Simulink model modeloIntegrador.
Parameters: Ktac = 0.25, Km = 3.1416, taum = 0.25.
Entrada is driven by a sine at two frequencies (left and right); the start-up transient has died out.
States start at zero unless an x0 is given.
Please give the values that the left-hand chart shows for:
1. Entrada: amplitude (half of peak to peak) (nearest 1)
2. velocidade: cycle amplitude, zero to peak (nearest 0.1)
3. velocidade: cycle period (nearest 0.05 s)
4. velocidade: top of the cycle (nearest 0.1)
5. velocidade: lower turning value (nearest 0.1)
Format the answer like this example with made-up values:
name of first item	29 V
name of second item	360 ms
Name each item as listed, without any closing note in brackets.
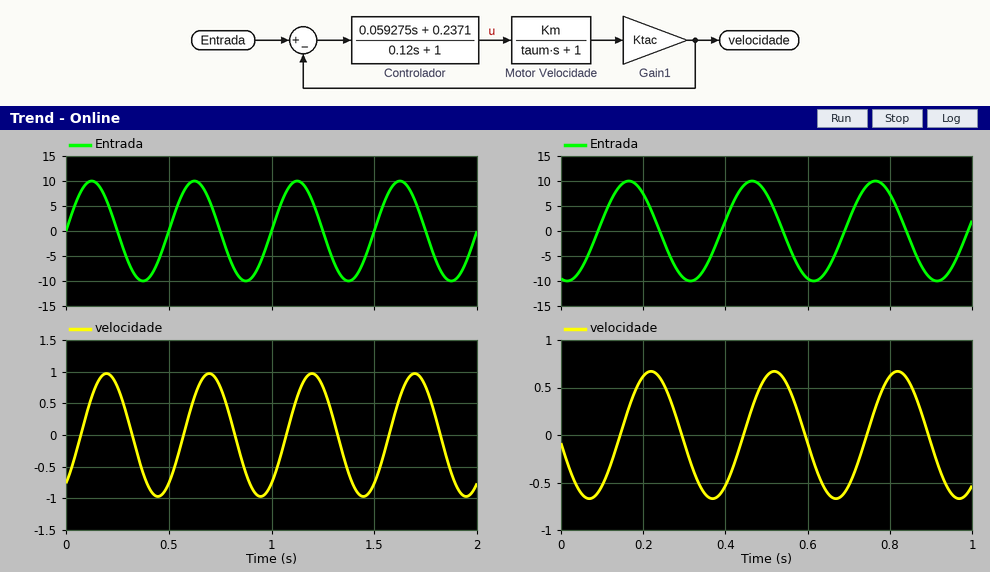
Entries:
Entrada: amplitude (half of peak to peak)	10
velocidade: cycle amplitude, zero to peak	1.0
velocidade: cycle period	0.50 s
velocidade: top of the cycle	1.0
velocidade: lower turning value	-1.0
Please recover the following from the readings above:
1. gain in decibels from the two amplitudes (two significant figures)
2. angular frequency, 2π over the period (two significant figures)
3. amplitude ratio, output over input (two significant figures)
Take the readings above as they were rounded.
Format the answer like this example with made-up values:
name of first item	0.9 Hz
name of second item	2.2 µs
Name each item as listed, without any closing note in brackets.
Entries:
gain in decibels from the two amplitudes	-20 dB
angular frequency, 2π over the period	13 rad/s
amplitude ratio, output over input	0.10
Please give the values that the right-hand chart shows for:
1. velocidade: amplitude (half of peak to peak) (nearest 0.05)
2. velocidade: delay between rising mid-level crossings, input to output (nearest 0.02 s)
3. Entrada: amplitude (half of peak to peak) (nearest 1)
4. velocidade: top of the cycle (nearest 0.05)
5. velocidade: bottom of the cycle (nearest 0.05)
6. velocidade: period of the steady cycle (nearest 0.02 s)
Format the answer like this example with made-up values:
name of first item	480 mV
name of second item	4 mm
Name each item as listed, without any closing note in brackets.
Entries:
velocidade: amplitude (half of peak to peak)	0.65
velocidade: delay between rising mid-level crossings, input to output	0.06 s
Entrada: amplitude (half of peak to peak)	10
velocidade: top of the cycle	0.65
velocidade: bottom of the cycle	-0.65
velocidade: period of the steady cycle	0.30 s
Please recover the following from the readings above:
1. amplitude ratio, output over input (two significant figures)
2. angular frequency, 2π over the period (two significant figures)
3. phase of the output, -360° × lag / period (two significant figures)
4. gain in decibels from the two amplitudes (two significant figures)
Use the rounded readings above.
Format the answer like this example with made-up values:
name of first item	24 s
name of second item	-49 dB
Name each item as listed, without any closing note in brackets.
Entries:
amplitude ratio, output over input	0.065
angular frequency, 2π over the period	21 rad/s
phase of the output, -360° × lag / period	-72°
gain in decibels from the two amplitudes	-24 dB
